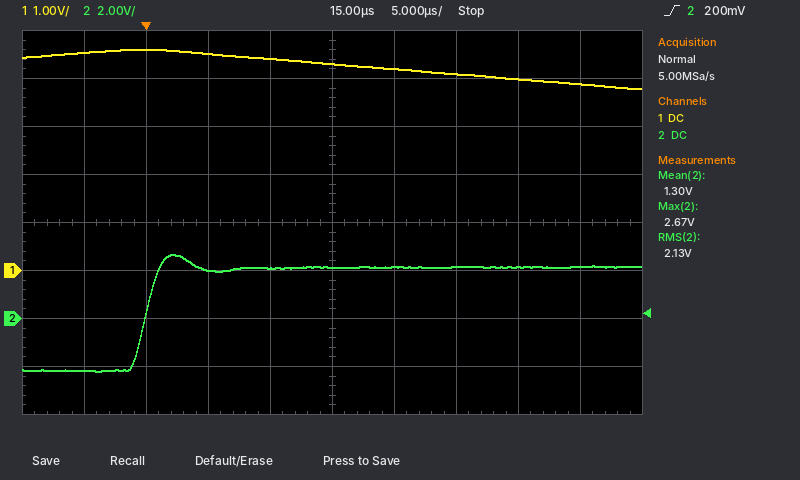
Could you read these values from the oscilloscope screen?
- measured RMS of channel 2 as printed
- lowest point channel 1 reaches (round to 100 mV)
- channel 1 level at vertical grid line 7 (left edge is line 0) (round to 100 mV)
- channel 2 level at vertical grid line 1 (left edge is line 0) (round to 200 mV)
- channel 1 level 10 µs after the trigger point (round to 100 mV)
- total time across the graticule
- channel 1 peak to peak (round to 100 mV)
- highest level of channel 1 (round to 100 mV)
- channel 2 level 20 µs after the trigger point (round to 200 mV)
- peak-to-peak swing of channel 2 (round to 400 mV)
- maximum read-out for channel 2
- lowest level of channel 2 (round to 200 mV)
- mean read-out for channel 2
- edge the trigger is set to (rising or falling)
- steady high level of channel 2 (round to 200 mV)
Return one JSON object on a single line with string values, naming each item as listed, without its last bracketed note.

{"measured RMS of channel 2 as printed": "2.13 V", "lowest point channel 1 reaches": "3.8 V", "channel 1 level at vertical grid line 7 (left edge is line 0)": "4.1 V", "channel 2 level at vertical grid line 1 (left edge is line 0)": "-2.2 V", "channel 1 level 10 µs after the trigger point": "4.4 V", "total time across the graticule": "50 µs", "channel 1 peak to peak": "800 mV", "highest level of channel 1": "4.6 V", "channel 2 level 20 µs after the trigger point": "2.2 V", "peak-to-peak swing of channel 2": "4.8 V", "maximum read-out for channel 2": "2.67 V", "lowest level of channel 2": "-2.2 V", "mean read-out for channel 2": "1.30 V", "edge the trigger is set to": "rising", "steady high level of channel 2": "2.2 V"}
